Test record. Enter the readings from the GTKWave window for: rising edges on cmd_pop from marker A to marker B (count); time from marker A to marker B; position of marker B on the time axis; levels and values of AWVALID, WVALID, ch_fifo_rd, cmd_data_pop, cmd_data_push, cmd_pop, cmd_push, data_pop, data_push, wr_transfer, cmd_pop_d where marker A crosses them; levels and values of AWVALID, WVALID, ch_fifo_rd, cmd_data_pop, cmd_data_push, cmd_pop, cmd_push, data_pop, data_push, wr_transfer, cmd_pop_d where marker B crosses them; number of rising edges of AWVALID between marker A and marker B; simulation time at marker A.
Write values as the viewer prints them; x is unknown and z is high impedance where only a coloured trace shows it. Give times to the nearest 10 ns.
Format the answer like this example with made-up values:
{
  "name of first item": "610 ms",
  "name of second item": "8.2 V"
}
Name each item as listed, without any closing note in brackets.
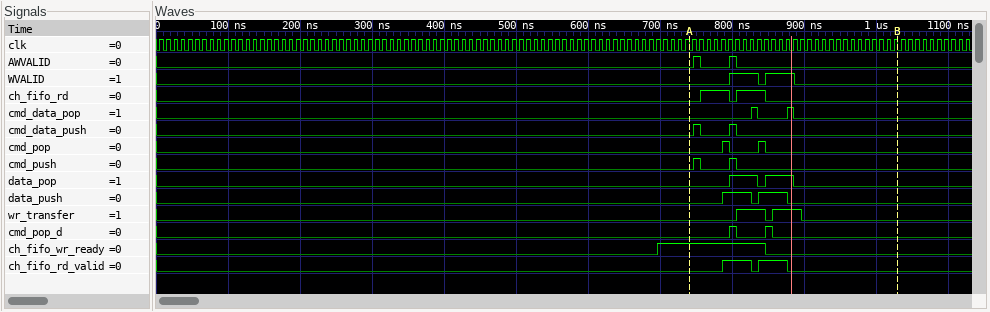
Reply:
{
  "rising edges on cmd_pop from marker A to marker B": "2",
  "time from marker A to marker B": "290 ns",
  "position of marker B on the time axis": "1030 ns",
  "levels and values of AWVALID, WVALID, ch_fifo_rd, cmd_data_pop, cmd_data_push, cmd_pop, cmd_push, data_pop, data_push, wr_transfer, cmd_pop_d where marker A crosses them": "AWVALID=0, WVALID=0, ch_fifo_rd=0, cmd_data_pop=0, cmd_data_push=0, cmd_pop=0, cmd_push=0, data_pop=0, data_push=0, wr_transfer=0, cmd_pop_d=0",
  "levels and values of AWVALID, WVALID, ch_fifo_rd, cmd_data_pop, cmd_data_push, cmd_pop, cmd_push, data_pop, data_push, wr_transfer, cmd_pop_d where marker B crosses them": "AWVALID=0, WVALID=0, ch_fifo_rd=0, cmd_data_pop=0, cmd_data_push=0, cmd_pop=0, cmd_push=0, data_pop=0, data_push=0, wr_transfer=0, cmd_pop_d=0",
  "number of rising edges of AWVALID between marker A and marker B": "2",
  "simulation time at marker A": "740 ns"
}
